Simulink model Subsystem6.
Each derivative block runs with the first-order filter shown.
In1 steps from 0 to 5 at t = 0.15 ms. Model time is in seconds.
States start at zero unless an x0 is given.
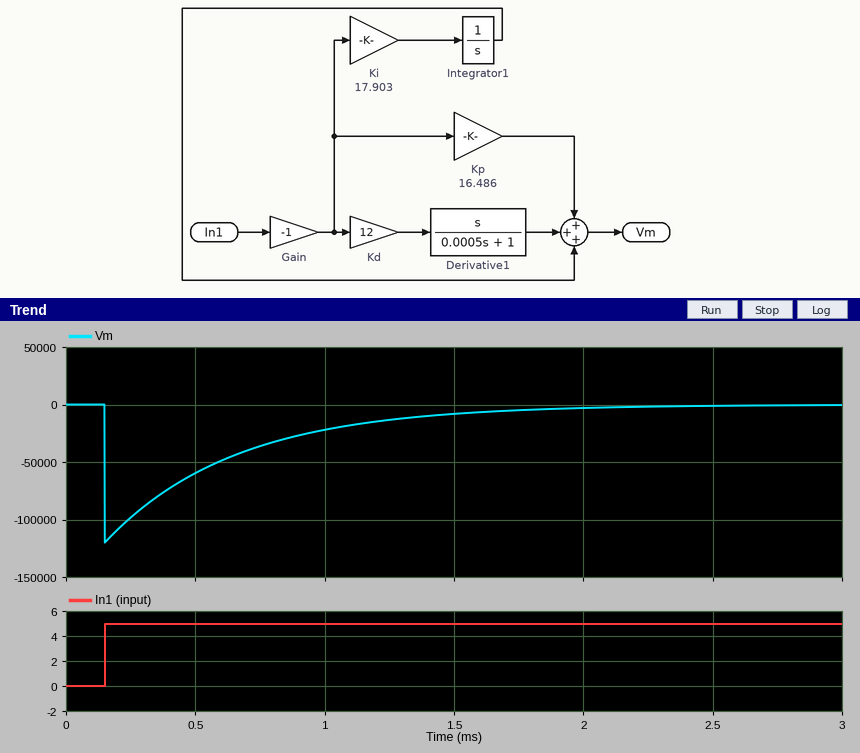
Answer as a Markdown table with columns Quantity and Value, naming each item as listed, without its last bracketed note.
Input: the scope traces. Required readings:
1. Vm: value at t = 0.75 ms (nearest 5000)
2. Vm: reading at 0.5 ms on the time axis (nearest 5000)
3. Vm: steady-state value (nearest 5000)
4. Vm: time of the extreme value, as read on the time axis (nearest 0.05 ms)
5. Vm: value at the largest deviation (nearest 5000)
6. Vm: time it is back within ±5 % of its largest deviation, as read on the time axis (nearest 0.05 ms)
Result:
| Quantity | Value |
|---|---|
| Vm: value at t = 0.75 ms | -35000 |
| Vm: reading at 0.5 ms on the time axis | -60000 |
| Vm: steady-state value | 0 |
| Vm: time of the extreme value, as read on the time axis | 0.15 ms |
| Vm: value at the largest deviation | -120000 |
| Vm: time it is back within ±5 % of its largest deviation, as read on the time axis | 1.65 ms |
